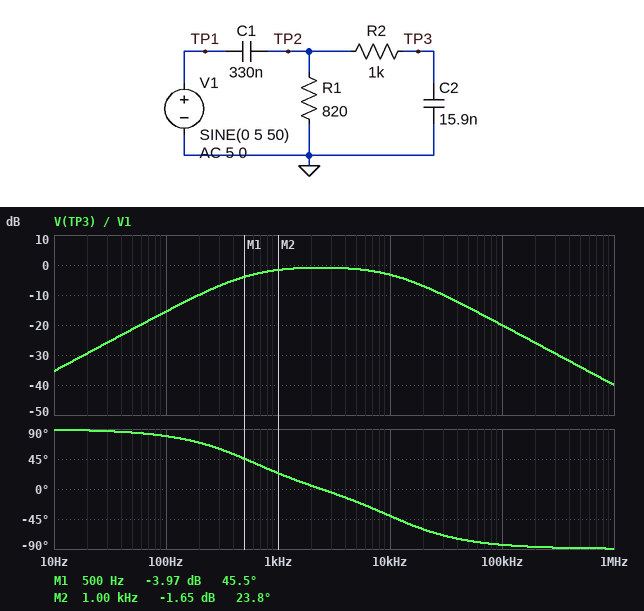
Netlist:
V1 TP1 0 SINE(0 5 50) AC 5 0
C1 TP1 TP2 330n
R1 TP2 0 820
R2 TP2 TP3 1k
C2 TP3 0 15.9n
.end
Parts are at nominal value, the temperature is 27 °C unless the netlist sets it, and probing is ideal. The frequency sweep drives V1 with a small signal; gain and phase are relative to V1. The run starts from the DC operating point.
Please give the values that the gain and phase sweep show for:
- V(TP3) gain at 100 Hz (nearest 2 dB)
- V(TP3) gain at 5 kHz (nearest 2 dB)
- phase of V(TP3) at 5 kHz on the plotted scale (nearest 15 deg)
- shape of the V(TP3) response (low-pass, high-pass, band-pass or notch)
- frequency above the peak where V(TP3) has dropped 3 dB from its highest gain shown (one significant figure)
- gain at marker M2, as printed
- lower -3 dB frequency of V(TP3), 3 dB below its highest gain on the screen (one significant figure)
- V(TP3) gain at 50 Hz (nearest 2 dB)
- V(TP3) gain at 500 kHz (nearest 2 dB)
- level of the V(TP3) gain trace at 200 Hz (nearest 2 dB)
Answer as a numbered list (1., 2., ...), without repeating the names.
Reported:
1. -16 dB
2. -2 dB
3. -15 deg
4. band-pass
5. 10 kHz
6. -1.65 dB
7. 500 Hz
8. -22 dB
9. -34 dB
10. -10 dB
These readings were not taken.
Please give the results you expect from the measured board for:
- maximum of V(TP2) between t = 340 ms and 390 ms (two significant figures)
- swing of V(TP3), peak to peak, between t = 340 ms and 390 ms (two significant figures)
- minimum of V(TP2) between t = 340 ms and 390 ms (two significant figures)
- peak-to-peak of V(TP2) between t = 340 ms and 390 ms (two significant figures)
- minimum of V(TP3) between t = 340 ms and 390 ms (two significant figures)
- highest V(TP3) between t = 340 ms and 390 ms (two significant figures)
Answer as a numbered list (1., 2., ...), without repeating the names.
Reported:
1. 420 mV
2. 850 mV
3. -420 mV
4. 850 mV
5. -420 mV
6. 420 mV
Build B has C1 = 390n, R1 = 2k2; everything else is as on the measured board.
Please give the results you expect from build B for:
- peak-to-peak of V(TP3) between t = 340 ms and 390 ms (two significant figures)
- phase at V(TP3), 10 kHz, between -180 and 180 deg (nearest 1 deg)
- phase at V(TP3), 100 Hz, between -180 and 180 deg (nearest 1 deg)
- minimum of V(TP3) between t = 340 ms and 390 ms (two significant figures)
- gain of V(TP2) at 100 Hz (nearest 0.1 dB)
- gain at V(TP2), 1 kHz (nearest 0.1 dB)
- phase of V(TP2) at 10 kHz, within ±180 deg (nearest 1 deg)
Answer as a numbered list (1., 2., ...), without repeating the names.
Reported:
1. 2.6 V
2. -43 deg
3. 60 deg
4. -1.3 V
5. -6.6 dB
6. -0.5 dB
7. 2 deg
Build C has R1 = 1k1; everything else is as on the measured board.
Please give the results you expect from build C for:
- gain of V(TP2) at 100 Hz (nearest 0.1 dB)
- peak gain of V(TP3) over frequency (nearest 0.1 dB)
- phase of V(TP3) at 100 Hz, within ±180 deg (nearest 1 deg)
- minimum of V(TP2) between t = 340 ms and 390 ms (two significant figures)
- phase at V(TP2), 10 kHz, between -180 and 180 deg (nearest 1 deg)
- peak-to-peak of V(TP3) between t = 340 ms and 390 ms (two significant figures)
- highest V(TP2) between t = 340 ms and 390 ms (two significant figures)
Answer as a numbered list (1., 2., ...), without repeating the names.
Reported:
1. -13.1 dB
2. -0.8 dB
3. 76 deg
4. -570 mV
5. 4 deg
6. 1.1 V
7. 570 mV
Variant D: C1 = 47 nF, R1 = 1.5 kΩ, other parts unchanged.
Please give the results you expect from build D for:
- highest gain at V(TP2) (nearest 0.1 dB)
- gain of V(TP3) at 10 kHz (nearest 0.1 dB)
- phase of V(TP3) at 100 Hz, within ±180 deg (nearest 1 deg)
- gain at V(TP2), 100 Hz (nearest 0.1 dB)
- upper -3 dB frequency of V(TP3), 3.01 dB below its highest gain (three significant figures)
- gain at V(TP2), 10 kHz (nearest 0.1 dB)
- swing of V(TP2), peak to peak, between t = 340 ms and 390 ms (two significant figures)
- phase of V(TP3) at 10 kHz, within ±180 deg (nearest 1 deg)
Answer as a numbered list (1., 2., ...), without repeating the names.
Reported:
1. 0 dB
2. -4.8 dB
3. 86 deg
4. -27.1 dB
5. 17.0 kHz
6. -1.8 dB
7. 220 mV
8. -26 deg
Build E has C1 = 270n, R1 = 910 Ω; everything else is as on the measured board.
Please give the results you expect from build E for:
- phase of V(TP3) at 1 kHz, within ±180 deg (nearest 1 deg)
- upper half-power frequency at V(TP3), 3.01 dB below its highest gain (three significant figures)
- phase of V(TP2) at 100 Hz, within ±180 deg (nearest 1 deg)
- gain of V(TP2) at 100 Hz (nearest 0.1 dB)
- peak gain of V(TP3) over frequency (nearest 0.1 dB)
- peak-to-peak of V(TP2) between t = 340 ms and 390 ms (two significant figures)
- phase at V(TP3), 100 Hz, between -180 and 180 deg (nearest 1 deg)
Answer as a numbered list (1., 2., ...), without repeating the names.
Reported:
1. 26 deg
2. 11.8 kHz
3. 81 deg
4. -16.3 dB
5. -1.0 dB
6. 770 mV
7. 80 deg
